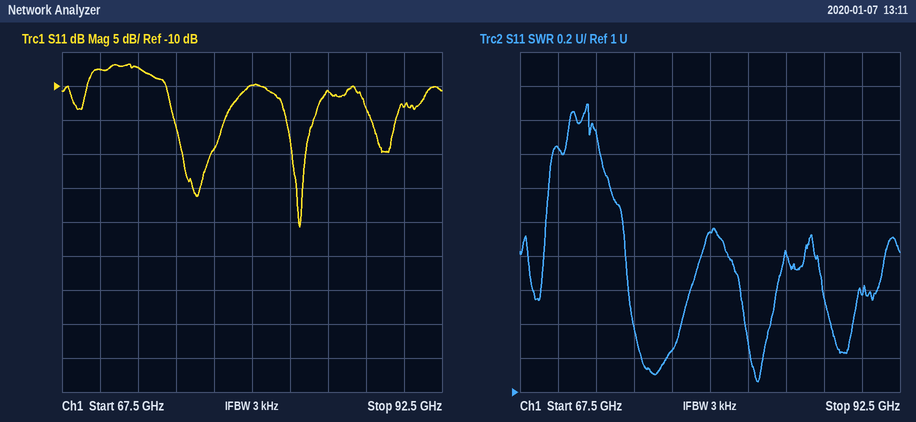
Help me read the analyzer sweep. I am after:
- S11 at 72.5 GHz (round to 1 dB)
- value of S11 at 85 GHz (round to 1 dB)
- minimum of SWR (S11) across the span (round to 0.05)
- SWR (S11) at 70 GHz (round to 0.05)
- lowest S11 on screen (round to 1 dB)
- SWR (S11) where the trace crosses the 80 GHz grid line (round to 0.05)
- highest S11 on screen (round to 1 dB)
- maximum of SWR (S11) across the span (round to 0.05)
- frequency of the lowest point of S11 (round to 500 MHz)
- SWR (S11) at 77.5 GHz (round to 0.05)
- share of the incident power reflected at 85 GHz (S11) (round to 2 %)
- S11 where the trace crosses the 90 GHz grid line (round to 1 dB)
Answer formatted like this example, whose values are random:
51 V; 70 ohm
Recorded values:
-7 dB; -11 dB; 1.05; 2.45; -31 dB; 1.95; -7 dB; 2.70; 83.0 GHz; 1.25; 8 %; -13 dB
